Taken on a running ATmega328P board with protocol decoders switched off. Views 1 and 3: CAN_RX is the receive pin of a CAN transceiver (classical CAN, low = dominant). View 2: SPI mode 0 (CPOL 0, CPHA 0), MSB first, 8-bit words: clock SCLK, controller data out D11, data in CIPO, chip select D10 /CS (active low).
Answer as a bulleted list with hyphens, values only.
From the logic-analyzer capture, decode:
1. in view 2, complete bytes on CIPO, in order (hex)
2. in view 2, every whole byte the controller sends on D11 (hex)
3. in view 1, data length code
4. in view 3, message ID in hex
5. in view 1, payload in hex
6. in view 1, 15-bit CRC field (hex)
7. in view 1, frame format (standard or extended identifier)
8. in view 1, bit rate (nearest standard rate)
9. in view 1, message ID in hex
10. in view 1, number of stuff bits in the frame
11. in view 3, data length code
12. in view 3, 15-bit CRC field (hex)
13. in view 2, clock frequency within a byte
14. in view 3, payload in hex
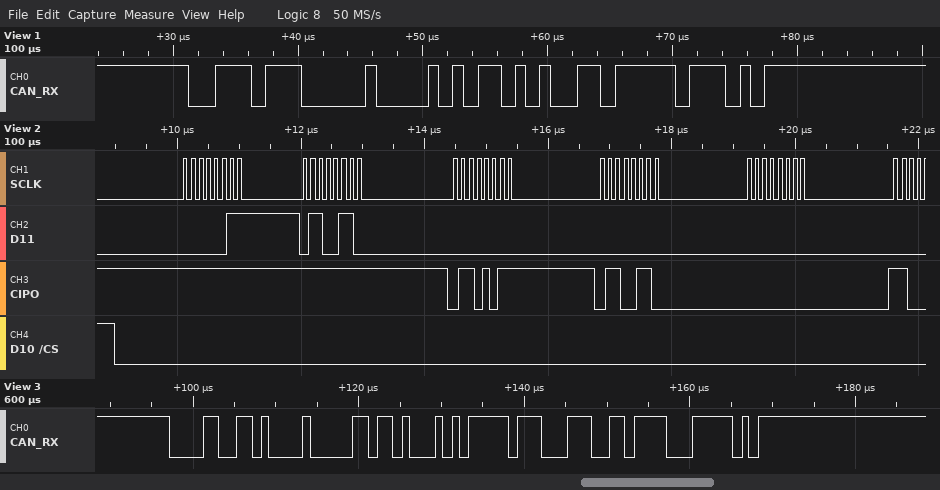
- FF FF 6B 66 00
- 03 66 00 00 00
- 1
- 0x0CD
- 5A
- 0x4DFE
- standard
- 1000 kbit/s
- 0x3B8
- 2
- 4
- 0x6F1F
- 8 MHz
- 16 8A FF 1C
